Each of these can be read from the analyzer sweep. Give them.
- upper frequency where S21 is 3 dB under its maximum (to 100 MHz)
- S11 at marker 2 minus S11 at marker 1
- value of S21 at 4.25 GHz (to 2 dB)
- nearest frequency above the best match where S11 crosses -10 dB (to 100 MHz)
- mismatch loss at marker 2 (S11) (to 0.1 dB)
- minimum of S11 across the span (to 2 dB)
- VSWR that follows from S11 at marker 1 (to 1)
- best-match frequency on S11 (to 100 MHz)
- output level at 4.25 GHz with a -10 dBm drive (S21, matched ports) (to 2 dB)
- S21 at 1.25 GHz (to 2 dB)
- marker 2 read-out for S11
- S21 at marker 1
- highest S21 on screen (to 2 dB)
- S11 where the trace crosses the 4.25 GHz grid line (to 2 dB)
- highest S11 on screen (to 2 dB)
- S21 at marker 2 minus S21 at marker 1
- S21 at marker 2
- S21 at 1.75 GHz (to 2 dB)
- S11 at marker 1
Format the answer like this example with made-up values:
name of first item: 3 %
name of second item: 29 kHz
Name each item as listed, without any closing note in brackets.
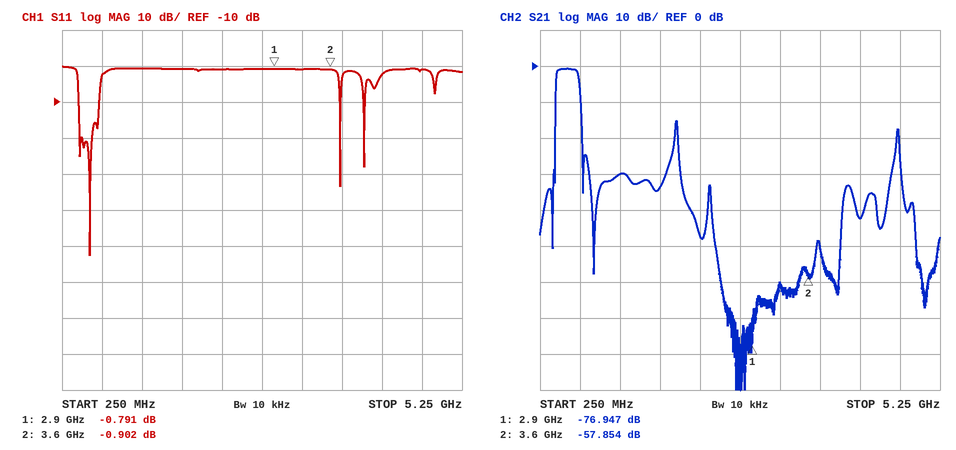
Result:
upper frequency where S21 is 3 dB under its maximum: 700 MHz
S11 at marker 2 minus S11 at marker 1: -0.111 dB
value of S21 at 4.25 GHz: -42 dB
nearest frequency above the best match where S11 crosses -10 dB: 700 MHz
mismatch loss at marker 2 (S11): 7.3 dB
minimum of S11 across the span: -52 dB
VSWR that follows from S11 at marker 1: 22
best-match frequency on S11: 600 MHz
output level at 4.25 GHz with a -10 dBm drive (S21, matched ports): -52 dBm
S21 at 1.25 GHz: -30 dB
marker 2 read-out for S11: -0.902 dB
S21 at marker 1: -76.947 dB
highest S21 on screen: 0 dB
S11 where the trace crosses the 4.25 GHz grid line: -2 dB
highest S11 on screen: 0 dB
S21 at marker 2 minus S21 at marker 1: 19.093 dB
S21 at marker 2: -57.854 dB
S21 at 1.75 GHz: -34 dB
S11 at marker 1: -0.791 dB
